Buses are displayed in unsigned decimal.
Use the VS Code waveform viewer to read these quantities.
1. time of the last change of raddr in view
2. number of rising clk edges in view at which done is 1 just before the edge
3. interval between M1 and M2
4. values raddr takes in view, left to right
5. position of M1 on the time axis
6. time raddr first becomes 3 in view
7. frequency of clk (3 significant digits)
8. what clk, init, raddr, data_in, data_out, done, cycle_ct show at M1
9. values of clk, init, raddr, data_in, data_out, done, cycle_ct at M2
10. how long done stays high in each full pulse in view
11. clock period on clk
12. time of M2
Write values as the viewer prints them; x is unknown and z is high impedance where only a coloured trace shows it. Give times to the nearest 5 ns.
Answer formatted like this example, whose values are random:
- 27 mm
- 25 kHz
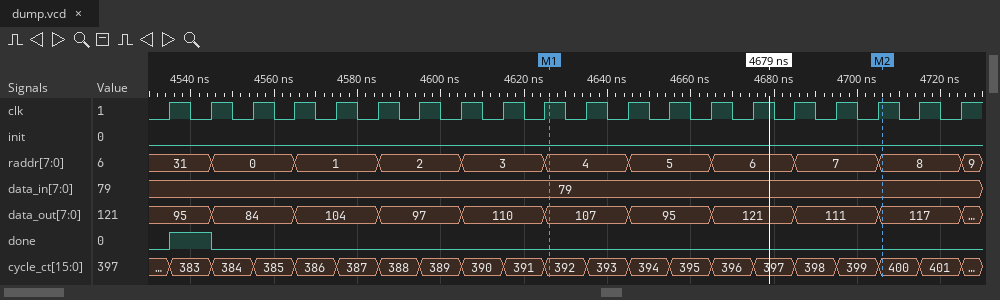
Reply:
- 4725 ns
- 1
- 80 ns
- 31, 0, 1, 2, 3, 4, 5, 6, 7, 8, 9
- 4625 ns
- 4605 ns
- 100 MHz
- clk=1, init=0, raddr=4, data_in=79, data_out=107, done=0, cycle_ct=392
- clk=1, init=0, raddr=8, data_in=79, data_out=117, done=0, cycle_ct=400
- 10 ns
- 10 ns
- 4705 ns
